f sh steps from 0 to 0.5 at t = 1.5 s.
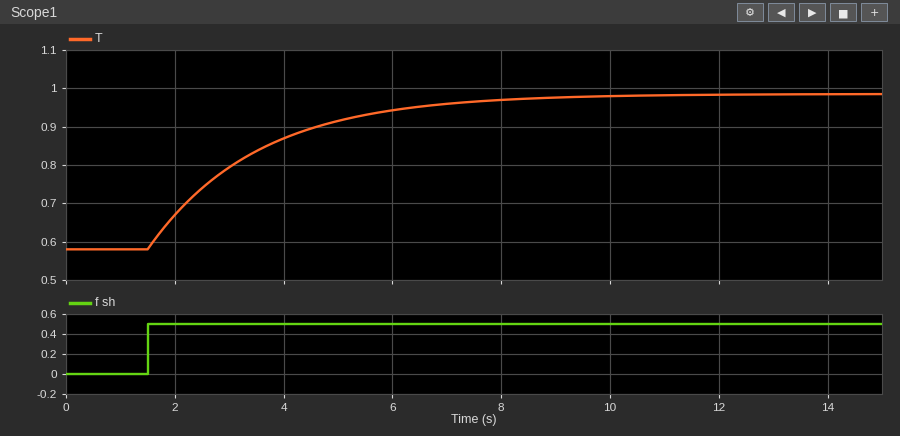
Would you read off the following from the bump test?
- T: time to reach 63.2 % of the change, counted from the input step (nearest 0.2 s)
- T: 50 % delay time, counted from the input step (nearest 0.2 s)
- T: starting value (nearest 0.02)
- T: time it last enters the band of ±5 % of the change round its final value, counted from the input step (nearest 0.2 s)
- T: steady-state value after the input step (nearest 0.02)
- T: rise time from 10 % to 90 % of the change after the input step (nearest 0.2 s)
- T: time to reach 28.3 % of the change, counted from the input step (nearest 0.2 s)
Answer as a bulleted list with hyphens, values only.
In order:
- 2.0 s
- 1.4 s
- 0.58
- 6.0 s
- 0.98
- 4.4 s
- 0.6 s
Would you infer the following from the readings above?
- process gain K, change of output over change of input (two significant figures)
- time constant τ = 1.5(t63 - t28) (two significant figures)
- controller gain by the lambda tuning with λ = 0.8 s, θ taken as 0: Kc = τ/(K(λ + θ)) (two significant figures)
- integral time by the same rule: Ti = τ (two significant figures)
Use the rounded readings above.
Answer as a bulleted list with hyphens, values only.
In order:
- 0.80
- 2.1 s
- 3.3
- 2.1 s
